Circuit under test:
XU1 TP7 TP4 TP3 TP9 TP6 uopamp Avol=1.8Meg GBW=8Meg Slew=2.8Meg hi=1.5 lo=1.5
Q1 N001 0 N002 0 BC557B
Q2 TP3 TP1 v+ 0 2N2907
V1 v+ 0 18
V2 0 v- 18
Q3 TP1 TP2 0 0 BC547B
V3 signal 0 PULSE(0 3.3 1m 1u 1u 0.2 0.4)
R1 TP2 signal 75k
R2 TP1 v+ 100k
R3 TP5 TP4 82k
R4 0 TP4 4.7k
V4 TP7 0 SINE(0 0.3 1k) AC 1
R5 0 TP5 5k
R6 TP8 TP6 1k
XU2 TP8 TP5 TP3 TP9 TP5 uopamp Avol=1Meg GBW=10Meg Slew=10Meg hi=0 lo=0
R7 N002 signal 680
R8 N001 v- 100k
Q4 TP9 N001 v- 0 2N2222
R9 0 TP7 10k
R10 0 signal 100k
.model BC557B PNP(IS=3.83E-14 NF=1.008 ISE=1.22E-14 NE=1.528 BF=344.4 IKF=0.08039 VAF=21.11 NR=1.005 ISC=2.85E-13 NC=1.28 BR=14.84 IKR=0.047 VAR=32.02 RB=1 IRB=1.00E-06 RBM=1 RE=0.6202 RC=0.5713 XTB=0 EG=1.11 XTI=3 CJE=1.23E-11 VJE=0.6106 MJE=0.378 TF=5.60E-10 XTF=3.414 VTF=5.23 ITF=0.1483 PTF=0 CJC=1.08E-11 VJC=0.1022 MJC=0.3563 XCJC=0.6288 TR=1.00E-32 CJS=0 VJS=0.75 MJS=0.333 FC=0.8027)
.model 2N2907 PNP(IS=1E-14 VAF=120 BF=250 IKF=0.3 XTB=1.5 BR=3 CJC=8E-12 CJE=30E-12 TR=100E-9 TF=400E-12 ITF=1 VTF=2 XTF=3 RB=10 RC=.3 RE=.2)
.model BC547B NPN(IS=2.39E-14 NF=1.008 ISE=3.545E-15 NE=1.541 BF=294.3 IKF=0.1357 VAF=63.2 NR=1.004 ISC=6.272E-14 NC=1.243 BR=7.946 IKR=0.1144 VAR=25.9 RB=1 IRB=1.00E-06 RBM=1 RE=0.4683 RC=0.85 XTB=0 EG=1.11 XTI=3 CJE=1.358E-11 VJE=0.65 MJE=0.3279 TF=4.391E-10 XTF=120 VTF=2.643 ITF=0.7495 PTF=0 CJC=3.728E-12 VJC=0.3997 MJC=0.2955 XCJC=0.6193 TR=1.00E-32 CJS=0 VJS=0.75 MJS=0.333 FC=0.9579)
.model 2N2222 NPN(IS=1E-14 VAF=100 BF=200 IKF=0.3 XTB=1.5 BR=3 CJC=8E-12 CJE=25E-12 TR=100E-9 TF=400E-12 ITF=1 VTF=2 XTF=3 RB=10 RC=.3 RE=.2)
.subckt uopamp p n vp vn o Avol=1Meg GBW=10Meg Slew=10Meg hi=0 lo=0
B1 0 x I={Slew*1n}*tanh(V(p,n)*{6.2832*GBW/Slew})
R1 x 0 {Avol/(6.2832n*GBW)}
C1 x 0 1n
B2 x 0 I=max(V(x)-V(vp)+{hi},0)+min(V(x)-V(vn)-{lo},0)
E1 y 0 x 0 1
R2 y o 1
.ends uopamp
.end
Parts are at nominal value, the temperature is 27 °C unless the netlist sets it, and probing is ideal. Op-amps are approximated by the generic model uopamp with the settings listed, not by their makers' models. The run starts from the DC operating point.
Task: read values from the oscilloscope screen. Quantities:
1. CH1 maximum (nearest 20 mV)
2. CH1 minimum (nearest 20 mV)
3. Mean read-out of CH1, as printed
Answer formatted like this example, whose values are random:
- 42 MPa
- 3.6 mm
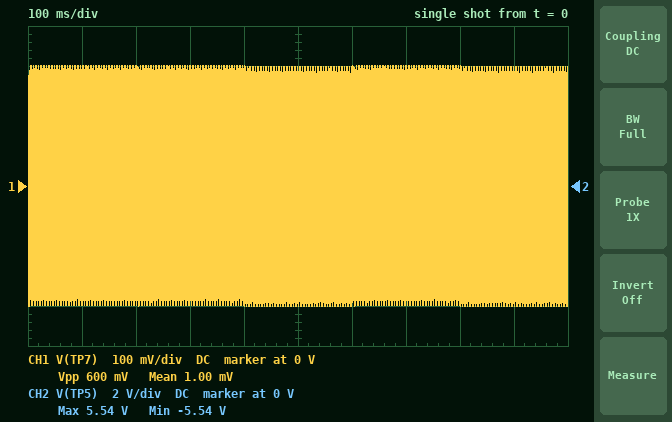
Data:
- 300 mV
- -300 mV
- 1.00 mV
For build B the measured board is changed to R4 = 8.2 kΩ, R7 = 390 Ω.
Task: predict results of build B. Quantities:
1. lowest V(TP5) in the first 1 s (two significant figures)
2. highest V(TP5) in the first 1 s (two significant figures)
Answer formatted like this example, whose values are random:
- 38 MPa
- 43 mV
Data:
- -3.3 V
- 3.3 V
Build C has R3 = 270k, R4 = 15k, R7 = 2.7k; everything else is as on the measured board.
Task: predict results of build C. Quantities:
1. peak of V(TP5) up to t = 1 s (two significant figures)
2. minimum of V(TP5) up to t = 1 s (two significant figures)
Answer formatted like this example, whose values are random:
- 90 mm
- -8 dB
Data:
- 5.7 V
- -5.7 V
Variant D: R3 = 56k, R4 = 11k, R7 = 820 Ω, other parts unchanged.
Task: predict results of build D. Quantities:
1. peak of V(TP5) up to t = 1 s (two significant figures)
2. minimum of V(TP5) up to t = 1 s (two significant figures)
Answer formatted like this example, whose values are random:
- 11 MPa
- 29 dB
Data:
- 1.8 V
- -1.8 V
